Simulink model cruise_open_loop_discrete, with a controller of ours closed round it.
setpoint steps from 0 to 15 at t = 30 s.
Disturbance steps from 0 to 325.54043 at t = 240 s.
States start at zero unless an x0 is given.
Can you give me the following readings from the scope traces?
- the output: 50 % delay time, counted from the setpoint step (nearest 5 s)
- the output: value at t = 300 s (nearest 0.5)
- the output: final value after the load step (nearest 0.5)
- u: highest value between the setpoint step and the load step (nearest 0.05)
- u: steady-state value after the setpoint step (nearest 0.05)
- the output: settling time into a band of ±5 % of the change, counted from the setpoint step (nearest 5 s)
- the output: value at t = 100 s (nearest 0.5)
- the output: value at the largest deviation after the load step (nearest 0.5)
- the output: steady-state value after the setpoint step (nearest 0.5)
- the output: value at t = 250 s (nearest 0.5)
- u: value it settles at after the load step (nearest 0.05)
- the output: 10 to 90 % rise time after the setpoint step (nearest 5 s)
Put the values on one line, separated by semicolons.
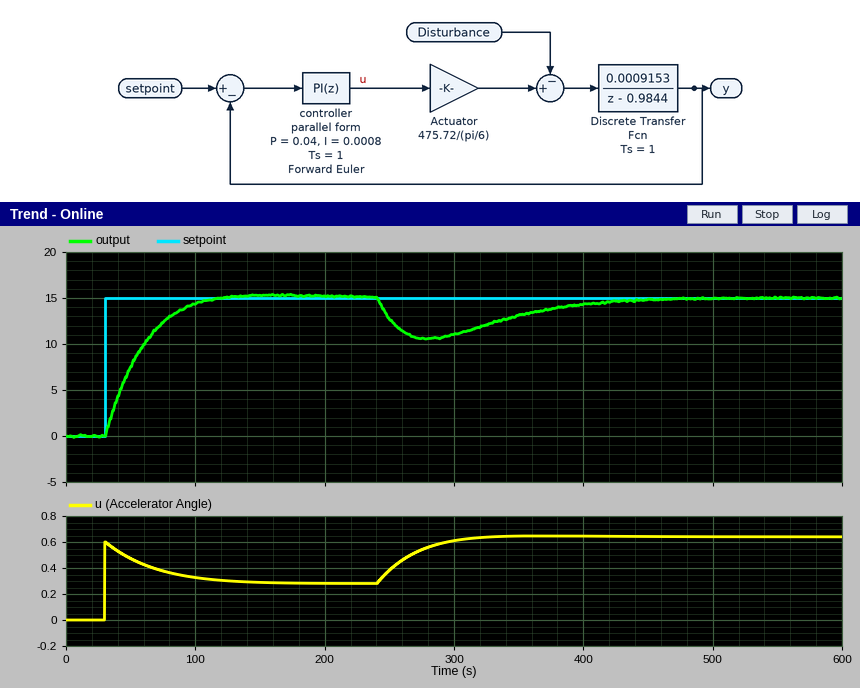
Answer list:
20 s; 11.0; 15.0; 0.60; 0.30; 70 s; 14.5; 10.5; 15.0; 12.5; 0.65; 55 s
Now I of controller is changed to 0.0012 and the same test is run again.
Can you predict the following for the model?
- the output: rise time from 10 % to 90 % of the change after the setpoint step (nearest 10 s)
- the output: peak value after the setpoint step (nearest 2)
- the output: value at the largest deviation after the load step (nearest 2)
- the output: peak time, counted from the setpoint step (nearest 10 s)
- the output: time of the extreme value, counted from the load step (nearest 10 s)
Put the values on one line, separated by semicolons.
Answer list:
40 s; 16; 10; 90 s; 30 s
